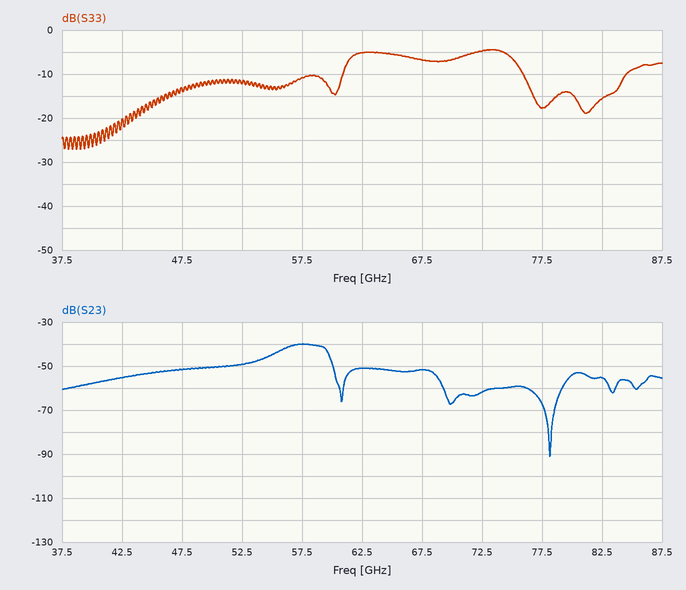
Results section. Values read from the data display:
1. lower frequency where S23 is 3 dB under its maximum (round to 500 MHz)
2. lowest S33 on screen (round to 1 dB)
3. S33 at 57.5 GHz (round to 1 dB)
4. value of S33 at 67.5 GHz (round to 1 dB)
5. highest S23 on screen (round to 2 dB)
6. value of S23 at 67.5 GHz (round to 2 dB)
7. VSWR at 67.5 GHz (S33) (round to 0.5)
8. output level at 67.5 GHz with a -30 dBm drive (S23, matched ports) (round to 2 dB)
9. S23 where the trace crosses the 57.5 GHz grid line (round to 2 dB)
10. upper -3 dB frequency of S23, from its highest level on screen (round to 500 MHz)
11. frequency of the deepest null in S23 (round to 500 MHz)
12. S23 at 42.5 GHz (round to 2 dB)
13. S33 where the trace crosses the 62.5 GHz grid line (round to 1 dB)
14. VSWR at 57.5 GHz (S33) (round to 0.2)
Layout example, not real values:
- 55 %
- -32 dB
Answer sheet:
- 55.5 GHz
- -27 dB
- -11 dB
- -7 dB
- -40 dB
- -52 dB
- 2.5
- -82 dBm
- -40 dB
- 59.5 GHz
- 78.0 GHz
- -56 dB
- -5 dB
- 1.8
